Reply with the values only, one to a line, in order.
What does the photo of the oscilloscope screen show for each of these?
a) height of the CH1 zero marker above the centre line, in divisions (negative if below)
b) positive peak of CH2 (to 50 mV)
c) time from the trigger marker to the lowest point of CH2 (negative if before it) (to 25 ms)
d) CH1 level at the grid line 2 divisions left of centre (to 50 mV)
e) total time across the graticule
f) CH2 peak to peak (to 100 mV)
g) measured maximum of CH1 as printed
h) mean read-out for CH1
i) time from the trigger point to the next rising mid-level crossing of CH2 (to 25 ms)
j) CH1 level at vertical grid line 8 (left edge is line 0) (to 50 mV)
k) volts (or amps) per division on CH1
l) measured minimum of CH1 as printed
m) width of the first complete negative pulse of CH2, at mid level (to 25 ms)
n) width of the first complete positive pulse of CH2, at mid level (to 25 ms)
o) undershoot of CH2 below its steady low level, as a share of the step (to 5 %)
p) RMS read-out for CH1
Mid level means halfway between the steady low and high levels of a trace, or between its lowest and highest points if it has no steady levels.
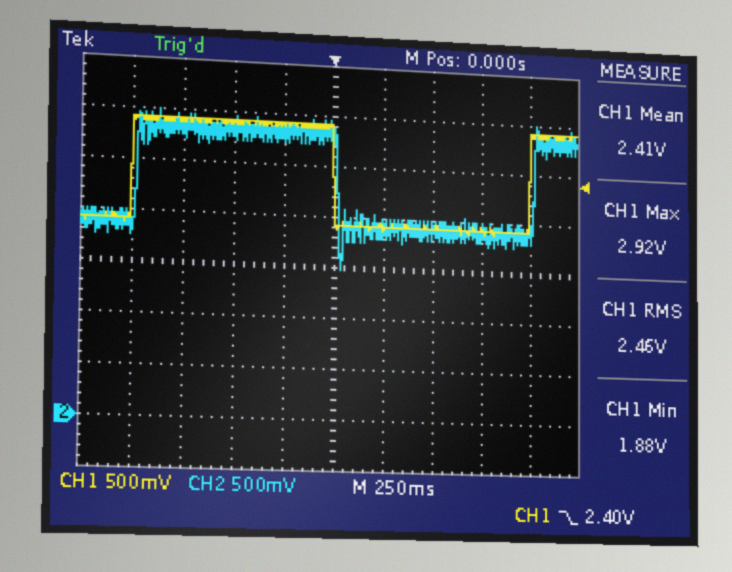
-3.0 div
3.00 V
+25 ms
2.90 V
2.5 s
1.50 V
2.92 V
2.41 V
1.025 s
1.90 V
500 mV
1.88 V
1.000 s
1.000 s
45 %
2.46 V
